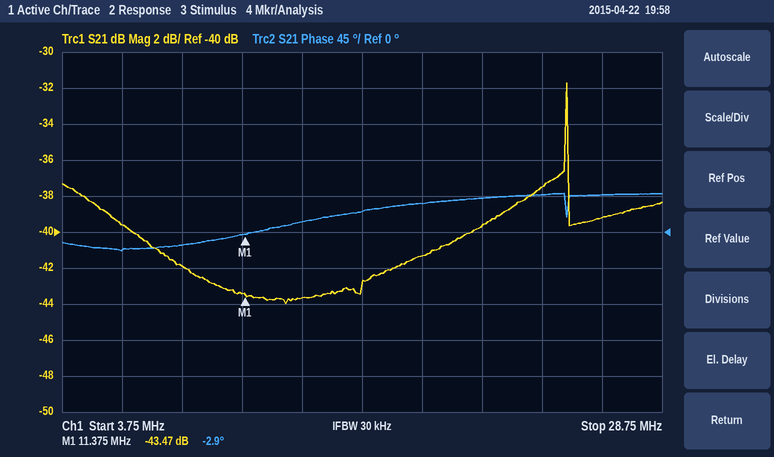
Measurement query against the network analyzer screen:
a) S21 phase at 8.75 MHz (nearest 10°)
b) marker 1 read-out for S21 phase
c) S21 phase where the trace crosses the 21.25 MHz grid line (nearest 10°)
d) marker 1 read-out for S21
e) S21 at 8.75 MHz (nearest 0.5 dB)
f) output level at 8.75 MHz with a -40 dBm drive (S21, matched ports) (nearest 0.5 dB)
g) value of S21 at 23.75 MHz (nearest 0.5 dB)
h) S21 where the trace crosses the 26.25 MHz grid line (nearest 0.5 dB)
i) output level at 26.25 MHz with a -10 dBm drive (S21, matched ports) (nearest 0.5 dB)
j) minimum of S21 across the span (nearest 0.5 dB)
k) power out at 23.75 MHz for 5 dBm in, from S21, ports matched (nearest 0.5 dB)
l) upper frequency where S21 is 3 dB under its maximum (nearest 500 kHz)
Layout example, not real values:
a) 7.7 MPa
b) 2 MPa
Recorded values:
a) -20°
b) -2.9°
c) 40°
d) -43.47 dB
e) -42.0 dB
f) -82.0 dBm
g) -37.5 dB
h) -39.0 dB
i) -49.0 dBm
j) -44.0 dB
k) -32.5 dBm
l) 25.0 MHz
